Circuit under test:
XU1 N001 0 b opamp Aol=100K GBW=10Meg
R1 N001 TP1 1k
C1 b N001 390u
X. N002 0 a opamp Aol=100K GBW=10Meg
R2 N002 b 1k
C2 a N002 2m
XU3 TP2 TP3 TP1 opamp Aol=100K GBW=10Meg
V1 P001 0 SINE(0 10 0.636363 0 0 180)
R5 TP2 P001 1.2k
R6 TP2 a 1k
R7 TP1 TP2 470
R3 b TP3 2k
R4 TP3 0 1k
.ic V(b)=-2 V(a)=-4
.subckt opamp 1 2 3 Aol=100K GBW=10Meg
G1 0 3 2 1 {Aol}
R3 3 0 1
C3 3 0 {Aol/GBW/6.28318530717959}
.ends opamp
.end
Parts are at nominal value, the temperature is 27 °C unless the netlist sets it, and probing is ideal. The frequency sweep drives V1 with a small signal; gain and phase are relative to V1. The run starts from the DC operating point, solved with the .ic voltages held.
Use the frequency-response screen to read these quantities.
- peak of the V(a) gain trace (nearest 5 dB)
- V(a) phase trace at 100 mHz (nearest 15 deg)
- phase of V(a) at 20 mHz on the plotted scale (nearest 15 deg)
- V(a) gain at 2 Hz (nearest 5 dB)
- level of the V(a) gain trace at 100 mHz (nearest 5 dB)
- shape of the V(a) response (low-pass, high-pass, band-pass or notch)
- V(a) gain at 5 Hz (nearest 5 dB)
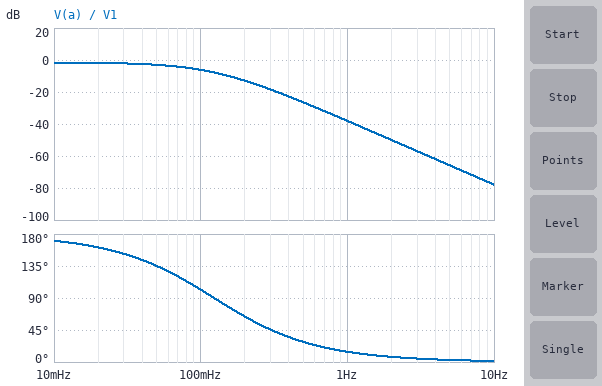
0 dB
105 deg
165 deg
-50 dB
-5 dB
low-pass
-65 dB
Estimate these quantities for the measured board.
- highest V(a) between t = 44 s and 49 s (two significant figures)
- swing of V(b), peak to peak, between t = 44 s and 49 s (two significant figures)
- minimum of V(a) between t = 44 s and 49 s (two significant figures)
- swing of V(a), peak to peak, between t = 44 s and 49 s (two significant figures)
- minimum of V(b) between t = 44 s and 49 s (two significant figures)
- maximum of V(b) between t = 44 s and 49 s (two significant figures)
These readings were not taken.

300 mV
4.8 V
-300 mV
600 mV
-2.4 V
2.4 V
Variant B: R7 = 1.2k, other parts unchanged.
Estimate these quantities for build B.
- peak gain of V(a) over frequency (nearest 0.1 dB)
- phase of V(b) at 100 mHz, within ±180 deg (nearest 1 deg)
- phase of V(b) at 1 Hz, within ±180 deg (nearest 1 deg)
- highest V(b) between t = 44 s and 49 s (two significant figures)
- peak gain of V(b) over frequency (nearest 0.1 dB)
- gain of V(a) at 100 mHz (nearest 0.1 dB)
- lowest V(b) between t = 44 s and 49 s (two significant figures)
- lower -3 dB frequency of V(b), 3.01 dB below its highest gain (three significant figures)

-1.6 dB
34 deg
-66 deg
5.7 V
-0.6 dB
-4.1 dB
-5.7 V
76.2 mHz
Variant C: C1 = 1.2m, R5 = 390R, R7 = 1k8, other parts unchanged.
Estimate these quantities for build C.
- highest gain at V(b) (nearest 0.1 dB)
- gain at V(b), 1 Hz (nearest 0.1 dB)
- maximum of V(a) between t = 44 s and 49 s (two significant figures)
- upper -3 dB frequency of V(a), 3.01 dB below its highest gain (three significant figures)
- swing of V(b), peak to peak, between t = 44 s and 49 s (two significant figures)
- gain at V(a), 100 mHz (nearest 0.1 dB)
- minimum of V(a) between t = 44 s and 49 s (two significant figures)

5.4 dB
-4.6 dB
1.1 V
69.7 mHz
18 V
3.1 dB
-1.1 V
